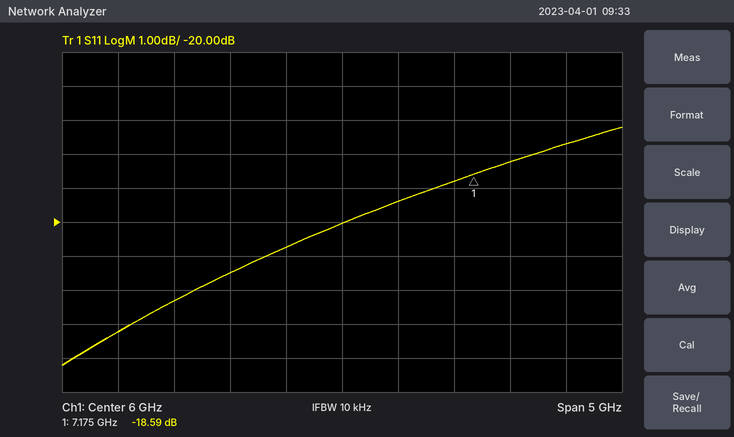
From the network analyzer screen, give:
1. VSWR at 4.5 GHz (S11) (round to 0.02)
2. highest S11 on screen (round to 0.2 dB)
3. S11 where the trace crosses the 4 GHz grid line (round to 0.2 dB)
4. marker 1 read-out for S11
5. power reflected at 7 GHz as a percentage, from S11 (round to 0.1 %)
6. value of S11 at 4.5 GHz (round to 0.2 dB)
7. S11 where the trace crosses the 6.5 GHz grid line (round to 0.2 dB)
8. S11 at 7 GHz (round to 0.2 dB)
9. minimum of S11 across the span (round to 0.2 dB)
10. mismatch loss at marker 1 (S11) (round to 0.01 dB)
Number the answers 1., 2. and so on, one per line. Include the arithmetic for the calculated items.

1. |Γ| = 10^(-22.4/20) = 0.0759; VSWR = (1 + 0.0759)/(1 − 0.0759) ≈ 1.16
2. -17.2 dB
3. -23.2 dB
4. -18.59 dB
5. 10^(-18.8/10) ≈ 1.3 %
6. -22.4 dB
7. -19.4 dB
8. -18.8 dB
9. -24.2 dB
10. −10 log10(1 − 10^(-18.59/10)) ≈ 0.06 dB
